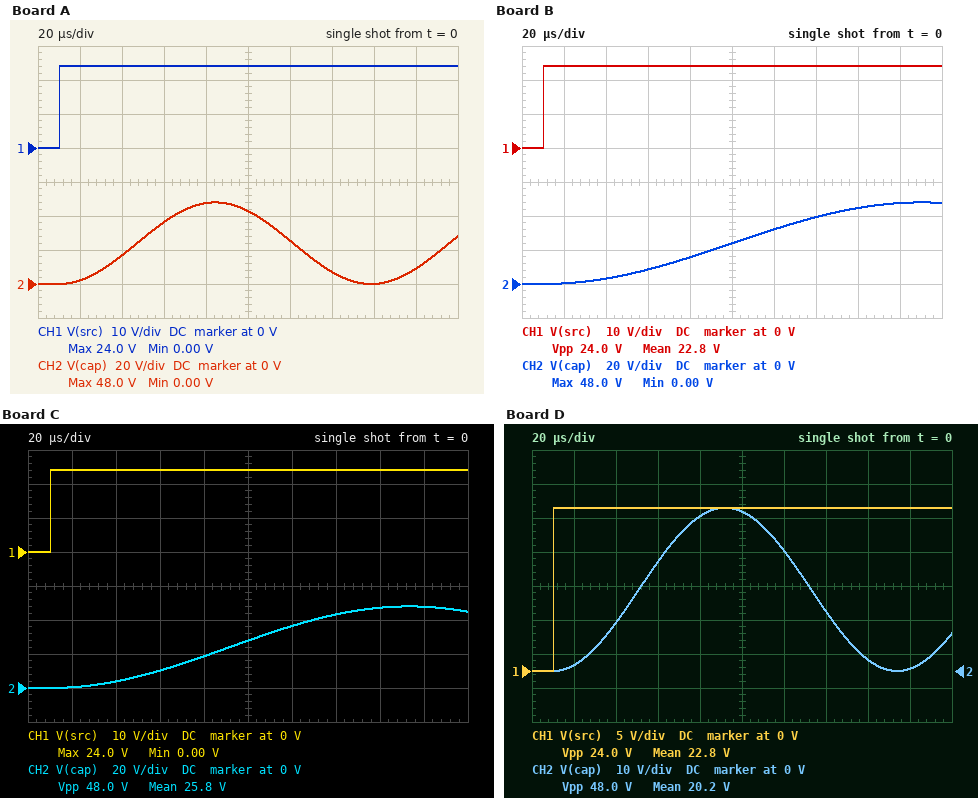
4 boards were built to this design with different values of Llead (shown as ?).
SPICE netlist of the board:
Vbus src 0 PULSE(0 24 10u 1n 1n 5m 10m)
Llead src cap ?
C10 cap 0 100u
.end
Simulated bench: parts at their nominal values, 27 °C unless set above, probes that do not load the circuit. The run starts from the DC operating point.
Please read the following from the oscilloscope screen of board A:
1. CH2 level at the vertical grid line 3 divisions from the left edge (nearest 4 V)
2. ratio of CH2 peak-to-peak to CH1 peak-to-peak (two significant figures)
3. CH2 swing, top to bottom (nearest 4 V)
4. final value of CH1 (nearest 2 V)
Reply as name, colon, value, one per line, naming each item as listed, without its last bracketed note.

CH2 level at the vertical grid line 3 divisions from the left edge: 36 V
ratio of CH2 peak-to-peak to CH1 peak-to-peak: 2.0
CH2 swing, top to bottom: 48 V
final value of CH1: 24 V
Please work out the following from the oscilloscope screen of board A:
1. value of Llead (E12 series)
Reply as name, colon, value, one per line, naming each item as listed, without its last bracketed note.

value of Llead: 5.6 µH
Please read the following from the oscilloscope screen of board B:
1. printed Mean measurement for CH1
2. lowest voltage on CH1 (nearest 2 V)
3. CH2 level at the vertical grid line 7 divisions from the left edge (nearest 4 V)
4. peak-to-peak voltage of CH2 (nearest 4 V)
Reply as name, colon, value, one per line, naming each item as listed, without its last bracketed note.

printed Mean measurement for CH1: 22.8 V
lowest voltage on CH1: 0 V
CH2 level at the vertical grid line 7 divisions from the left edge: 40 V
peak-to-peak voltage of CH2: 48 V
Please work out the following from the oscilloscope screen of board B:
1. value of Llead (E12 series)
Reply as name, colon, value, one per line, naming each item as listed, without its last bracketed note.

value of Llead: 33 µH
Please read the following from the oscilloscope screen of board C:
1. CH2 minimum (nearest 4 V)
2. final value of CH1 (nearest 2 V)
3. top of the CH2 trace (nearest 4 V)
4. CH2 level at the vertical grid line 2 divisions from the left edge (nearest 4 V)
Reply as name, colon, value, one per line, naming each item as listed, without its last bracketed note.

CH2 minimum: 0 V
final value of CH1: 24 V
top of the CH2 trace: 48 V
CH2 level at the vertical grid line 2 divisions from the left edge: 4 V
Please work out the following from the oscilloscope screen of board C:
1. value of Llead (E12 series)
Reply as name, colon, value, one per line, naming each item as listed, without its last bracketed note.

value of Llead: 27 µH
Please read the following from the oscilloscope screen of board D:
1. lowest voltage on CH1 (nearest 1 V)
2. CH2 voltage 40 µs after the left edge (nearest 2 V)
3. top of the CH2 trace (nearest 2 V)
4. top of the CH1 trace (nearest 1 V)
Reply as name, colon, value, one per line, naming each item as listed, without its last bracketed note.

lowest voltage on CH1: 0 V
CH2 voltage 40 µs after the left edge: 14 V
top of the CH2 trace: 48 V
top of the CH1 trace: 24 V
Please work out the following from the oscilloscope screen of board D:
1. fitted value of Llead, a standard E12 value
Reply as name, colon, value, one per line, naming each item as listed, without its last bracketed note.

fitted value of Llead, a standard E12 value: 6.8 µH
